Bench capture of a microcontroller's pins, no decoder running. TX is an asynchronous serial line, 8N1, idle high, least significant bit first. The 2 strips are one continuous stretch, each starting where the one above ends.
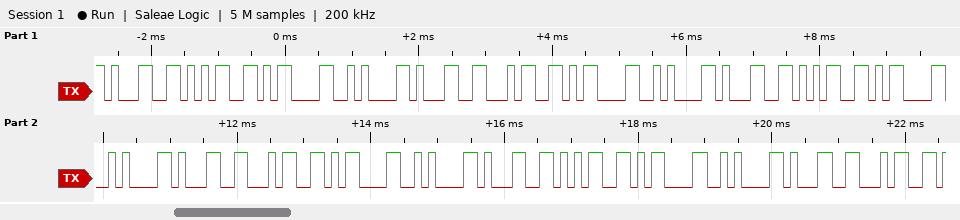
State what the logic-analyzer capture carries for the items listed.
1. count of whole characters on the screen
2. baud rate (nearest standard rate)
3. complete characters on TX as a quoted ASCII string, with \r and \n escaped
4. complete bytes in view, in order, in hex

22
9600 baud
"15\r\n14\r\n15\r\n14\r\n15\r\n14"
0x31 0x35 0x0D 0x0A 0x31 0x34 0x0D 0x0A 0x31 0x35 0x0D 0x0A 0x31 0x34 0x0D 0x0A 0x31 0x35 0x0D 0x0A 0x31 0x34
